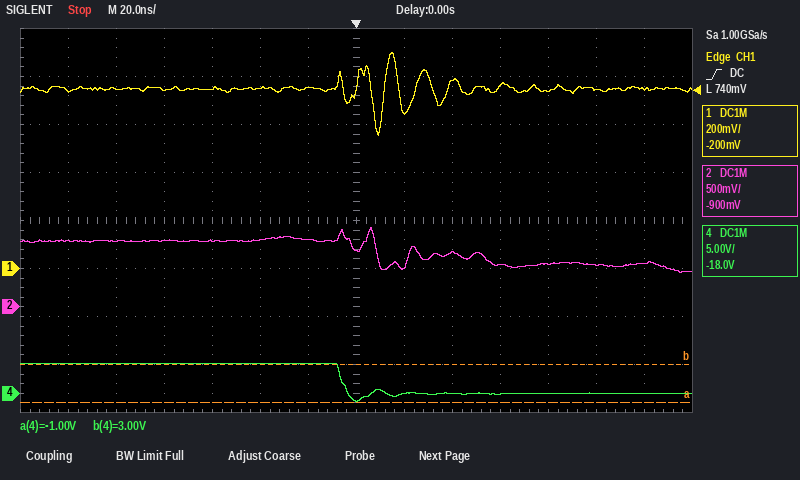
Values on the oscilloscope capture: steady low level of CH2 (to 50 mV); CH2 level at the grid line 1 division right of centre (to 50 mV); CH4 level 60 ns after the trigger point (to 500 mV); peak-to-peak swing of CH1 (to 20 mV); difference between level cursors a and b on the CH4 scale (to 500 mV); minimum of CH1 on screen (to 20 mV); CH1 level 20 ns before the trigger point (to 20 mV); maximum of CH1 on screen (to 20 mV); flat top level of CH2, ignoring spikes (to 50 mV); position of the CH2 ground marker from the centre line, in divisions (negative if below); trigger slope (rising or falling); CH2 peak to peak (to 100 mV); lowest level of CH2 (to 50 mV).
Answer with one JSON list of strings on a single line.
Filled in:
["450 mV", "400 mV", "0.0 V", "340 mV", "4.0 V", "560 mV", "760 mV", "900 mV", "700 mV", "-1.8 div", "rising", "500 mV", "350 mV"]
